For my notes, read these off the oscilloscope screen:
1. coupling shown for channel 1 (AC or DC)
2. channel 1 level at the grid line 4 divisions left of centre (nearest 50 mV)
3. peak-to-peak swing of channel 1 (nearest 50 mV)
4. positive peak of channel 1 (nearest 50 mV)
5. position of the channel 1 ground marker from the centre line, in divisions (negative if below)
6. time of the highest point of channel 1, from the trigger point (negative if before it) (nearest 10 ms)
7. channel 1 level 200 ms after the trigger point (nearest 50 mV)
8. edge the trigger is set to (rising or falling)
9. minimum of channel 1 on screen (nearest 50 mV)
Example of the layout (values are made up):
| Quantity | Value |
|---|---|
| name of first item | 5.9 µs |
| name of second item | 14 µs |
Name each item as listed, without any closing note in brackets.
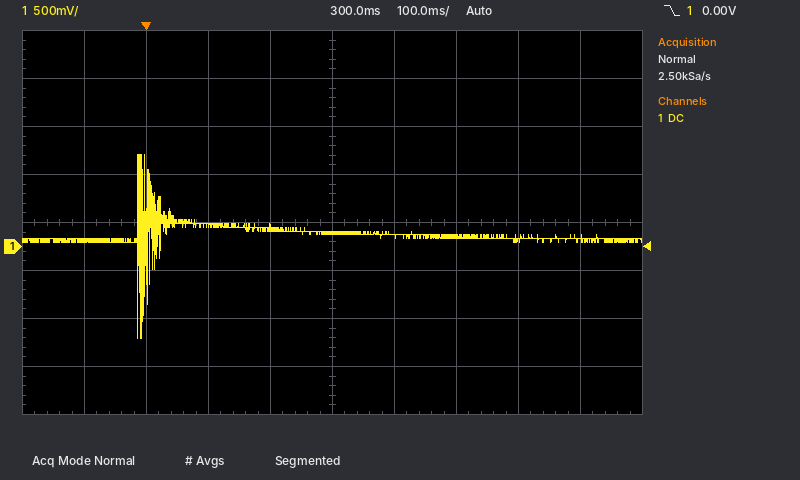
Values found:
| Quantity | Value |
|---|---|
| coupling shown for channel 1 | DC |
| channel 1 level at the grid line 4 divisions left of centre | 50 mV |
| peak-to-peak swing of channel 1 | 1.90 V |
| positive peak of channel 1 | 950 mV |
| position of the channel 1 ground marker from the centre line, in divisions | -0.5 div |
| time of the highest point of channel 1, from the trigger point (negative if before it) | -10 ms |
| channel 1 level 200 ms after the trigger point | 200 mV |
| edge the trigger is set to | falling |
| minimum of channel 1 on screen | -950 mV |
